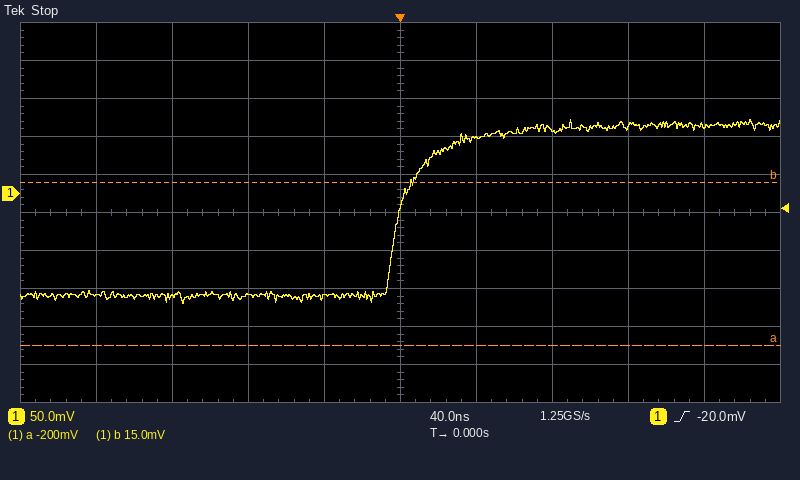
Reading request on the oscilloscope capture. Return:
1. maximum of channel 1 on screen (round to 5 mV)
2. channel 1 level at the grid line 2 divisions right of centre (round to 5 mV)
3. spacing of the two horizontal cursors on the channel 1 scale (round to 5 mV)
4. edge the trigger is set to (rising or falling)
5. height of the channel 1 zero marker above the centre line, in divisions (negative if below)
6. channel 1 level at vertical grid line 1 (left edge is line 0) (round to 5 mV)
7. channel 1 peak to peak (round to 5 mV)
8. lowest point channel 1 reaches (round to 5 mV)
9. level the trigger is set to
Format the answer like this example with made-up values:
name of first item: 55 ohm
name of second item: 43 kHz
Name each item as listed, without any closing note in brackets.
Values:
maximum of channel 1 on screen: 95 mV
channel 1 level at the grid line 2 divisions right of centre: 85 mV
spacing of the two horizontal cursors on the channel 1 scale: 215 mV
edge the trigger is set to: rising
height of the channel 1 zero marker above the centre line, in divisions: +0.5 div
channel 1 level at vertical grid line 1 (left edge is line 0): -135 mV
channel 1 peak to peak: 240 mV
lowest point channel 1 reaches: -145 mV
level the trigger is set to: -20.0 mV
